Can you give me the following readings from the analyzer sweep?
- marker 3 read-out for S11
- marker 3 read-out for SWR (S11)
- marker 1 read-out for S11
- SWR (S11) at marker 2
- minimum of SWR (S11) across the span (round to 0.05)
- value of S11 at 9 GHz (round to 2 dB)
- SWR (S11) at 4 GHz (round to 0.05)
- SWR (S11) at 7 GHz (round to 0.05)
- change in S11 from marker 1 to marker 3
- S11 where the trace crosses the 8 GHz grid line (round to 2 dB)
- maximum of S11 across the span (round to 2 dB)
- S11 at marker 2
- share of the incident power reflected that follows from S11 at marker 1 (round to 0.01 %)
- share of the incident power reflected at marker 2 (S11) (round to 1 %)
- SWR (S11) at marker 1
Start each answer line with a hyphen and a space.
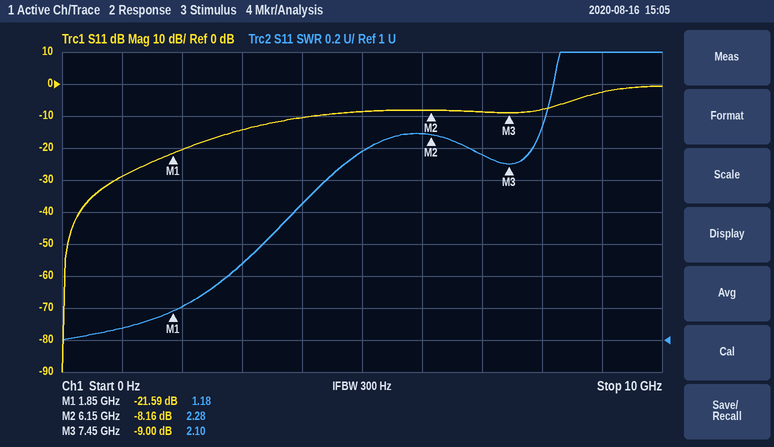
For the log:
- -9.00 dB
- 2.10
- -21.59 dB
- 2.28
- 1.00
- -2 dB
- 1.85
- 2.15
- 12.59 dB
- -8 dB
- 0 dB
- -8.16 dB
- 0.69 %
- 15 %
- 1.18
